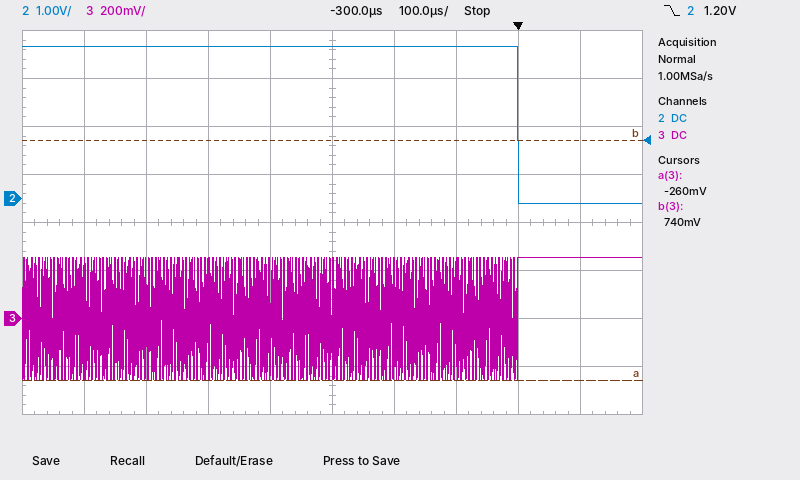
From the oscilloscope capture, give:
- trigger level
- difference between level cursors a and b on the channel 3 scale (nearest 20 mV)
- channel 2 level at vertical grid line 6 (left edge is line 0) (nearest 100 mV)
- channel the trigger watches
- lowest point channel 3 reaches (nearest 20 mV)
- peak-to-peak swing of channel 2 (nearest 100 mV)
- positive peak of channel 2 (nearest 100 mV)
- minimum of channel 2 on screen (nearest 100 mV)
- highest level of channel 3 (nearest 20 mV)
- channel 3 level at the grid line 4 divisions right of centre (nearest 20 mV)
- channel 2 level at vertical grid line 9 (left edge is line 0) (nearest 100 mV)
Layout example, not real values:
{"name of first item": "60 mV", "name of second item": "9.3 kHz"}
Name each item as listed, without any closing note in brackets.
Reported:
{"trigger level": "1.20 V", "difference between level cursors a and b on the channel 3 scale": "1.00 V", "channel 2 level at vertical grid line 6 (left edge is line 0)": "3.2 V", "channel the trigger watches": "channel 2", "lowest point channel 3 reaches": "-260 mV", "peak-to-peak swing of channel 2": "3.3 V", "positive peak of channel 2": "3.2 V", "minimum of channel 2 on screen": "-100 mV", "highest level of channel 3": "260 mV", "channel 3 level at the grid line 4 divisions right of centre": "260 mV", "channel 2 level at vertical grid line 9 (left edge is line 0)": "-100 mV"}
